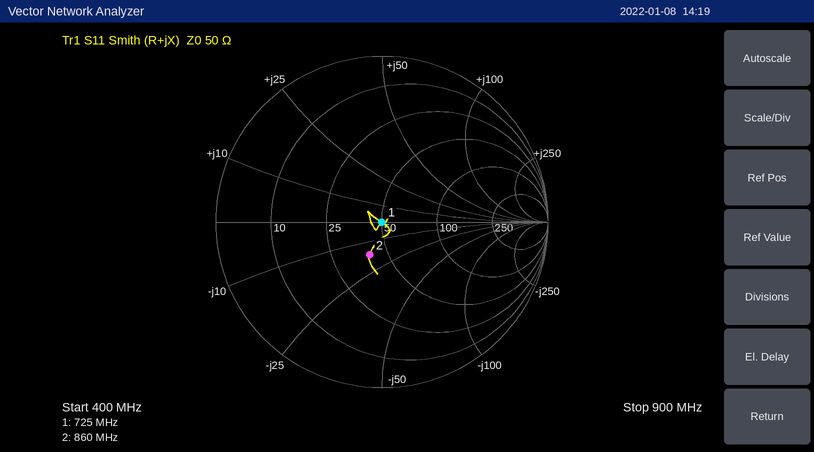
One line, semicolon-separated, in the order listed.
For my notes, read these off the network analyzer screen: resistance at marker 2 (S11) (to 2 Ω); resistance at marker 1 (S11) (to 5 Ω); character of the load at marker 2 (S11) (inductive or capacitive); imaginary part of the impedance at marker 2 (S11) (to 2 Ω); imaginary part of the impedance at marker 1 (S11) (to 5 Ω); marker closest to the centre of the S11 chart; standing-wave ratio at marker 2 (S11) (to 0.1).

40 Ω; 50 Ω; capacitive; -16 Ω; 0 Ω; marker 1; 1.5
